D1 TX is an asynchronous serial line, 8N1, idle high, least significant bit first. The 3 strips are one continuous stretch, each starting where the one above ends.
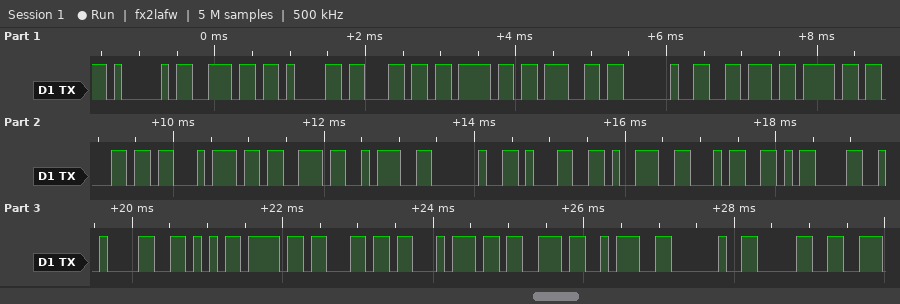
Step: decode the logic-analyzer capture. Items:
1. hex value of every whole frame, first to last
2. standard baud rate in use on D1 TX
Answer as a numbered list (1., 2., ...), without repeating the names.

1. 0x41 0x6E 0x61 0x6C 0x6F 0x67 0x20 0x76 0x6F 0x6C 0x74 0x73 0x3A 0x20 0x31 0x39 0x34 0x0D 0x0A 0x56 0x6F 0x6C 0x74 0x73 0x3A 0x20 0x30
2. 9600 baud
